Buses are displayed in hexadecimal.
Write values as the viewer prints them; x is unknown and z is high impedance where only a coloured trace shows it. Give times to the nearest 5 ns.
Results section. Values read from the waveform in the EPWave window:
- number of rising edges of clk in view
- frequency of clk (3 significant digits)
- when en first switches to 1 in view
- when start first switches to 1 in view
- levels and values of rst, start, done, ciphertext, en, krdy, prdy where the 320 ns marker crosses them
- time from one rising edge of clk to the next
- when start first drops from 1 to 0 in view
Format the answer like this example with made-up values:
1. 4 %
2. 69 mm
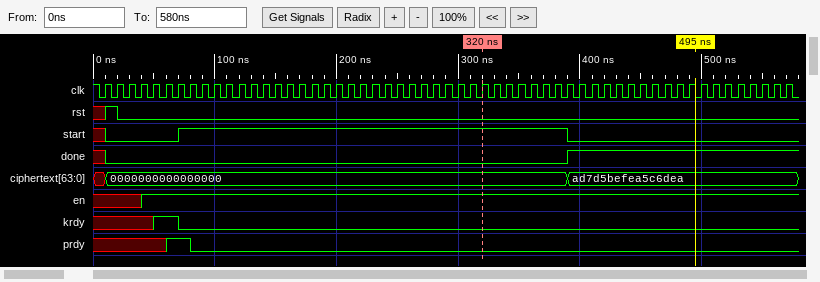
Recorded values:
1. 57
2. 100 MHz
3. 40 ns
4. 70 ns
5. rst=0, start=1, done=0, ciphertext=0000000000000000, en=1, krdy=0, prdy=0
6. 10 ns
7. 390 ns
